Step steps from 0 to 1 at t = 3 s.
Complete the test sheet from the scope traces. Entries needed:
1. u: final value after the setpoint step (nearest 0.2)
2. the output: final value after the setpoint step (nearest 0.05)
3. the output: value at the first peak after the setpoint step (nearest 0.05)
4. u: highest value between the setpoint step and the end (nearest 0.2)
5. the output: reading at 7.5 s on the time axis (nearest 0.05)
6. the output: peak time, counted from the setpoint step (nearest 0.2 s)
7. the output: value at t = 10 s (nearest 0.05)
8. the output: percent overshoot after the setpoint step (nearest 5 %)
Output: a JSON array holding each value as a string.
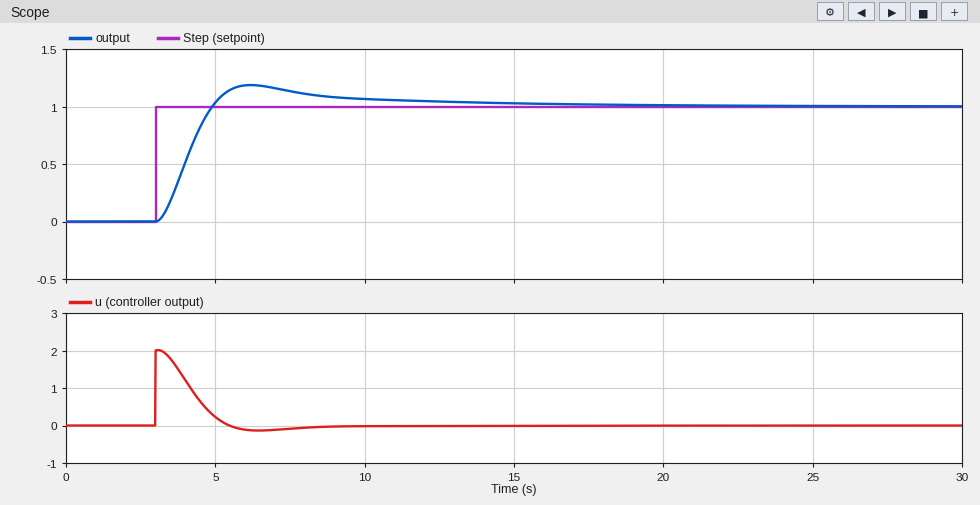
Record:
["0.0", "1.00", "1.20", "2.0", "1.15", "3.2 s", "1.05", "20 %"]
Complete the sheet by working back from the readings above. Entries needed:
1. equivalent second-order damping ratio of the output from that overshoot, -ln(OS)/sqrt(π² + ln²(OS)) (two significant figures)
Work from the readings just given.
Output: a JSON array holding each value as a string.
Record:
["0.46"]
